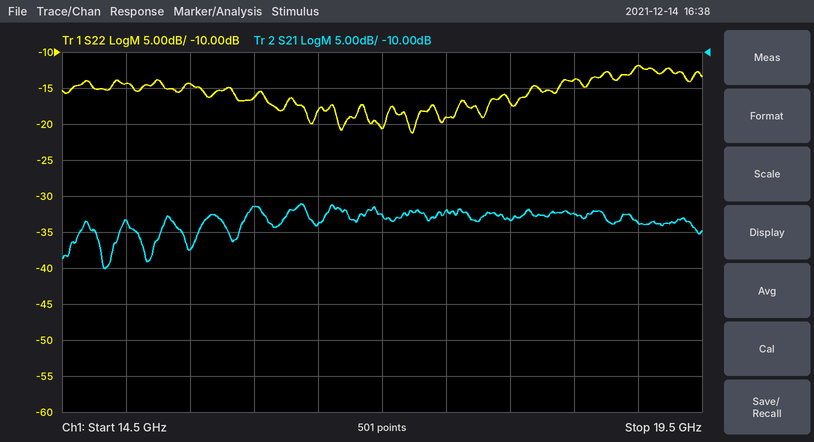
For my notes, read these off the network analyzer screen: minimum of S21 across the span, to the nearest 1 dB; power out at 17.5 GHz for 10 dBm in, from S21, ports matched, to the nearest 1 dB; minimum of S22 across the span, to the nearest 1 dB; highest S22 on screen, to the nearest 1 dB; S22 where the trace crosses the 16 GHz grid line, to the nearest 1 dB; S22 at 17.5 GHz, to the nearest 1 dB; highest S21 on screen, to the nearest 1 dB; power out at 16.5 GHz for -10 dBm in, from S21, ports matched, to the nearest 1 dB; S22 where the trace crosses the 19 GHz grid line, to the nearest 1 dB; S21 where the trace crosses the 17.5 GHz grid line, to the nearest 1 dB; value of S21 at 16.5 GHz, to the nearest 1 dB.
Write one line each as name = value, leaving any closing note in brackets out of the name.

minimum of S21 across the span, to the nearest 1 dB = -40 dB
power out at 17.5 GHz for 10 dBm in, from S21, ports matched, to the nearest 1 dB = -22 dBm
minimum of S22 across the span, to the nearest 1 dB = -21 dB
highest S22 on screen, to the nearest 1 dB = -12 dB
S22 where the trace crosses the 16 GHz grid line, to the nearest 1 dB = -16 dB
S22 at 17.5 GHz, to the nearest 1 dB = -19 dB
highest S21 on screen, to the nearest 1 dB = -31 dB
power out at 16.5 GHz for -10 dBm in, from S21, ports matched, to the nearest 1 dB = -44 dBm
S22 where the trace crosses the 19 GHz grid line, to the nearest 1 dB = -12 dB
S21 where the trace crosses the 17.5 GHz grid line, to the nearest 1 dB = -32 dB
value of S21 at 16.5 GHz, to the nearest 1 dB = -34 dB
